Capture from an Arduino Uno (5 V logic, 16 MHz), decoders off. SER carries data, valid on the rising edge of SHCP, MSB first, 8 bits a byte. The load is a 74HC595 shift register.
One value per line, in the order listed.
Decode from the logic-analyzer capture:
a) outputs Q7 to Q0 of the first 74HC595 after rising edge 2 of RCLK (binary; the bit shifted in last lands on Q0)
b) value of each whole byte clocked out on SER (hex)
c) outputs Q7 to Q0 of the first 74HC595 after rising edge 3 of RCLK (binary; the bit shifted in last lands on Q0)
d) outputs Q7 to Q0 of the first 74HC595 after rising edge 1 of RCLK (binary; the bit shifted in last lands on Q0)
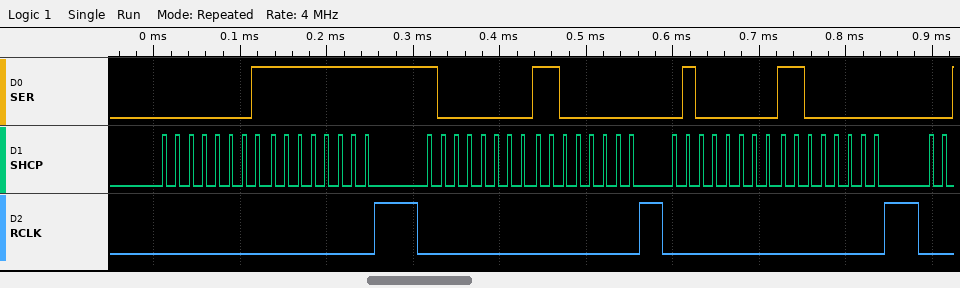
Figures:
11000000
01 FF 80 C0 40 C0
11000000
11111111
